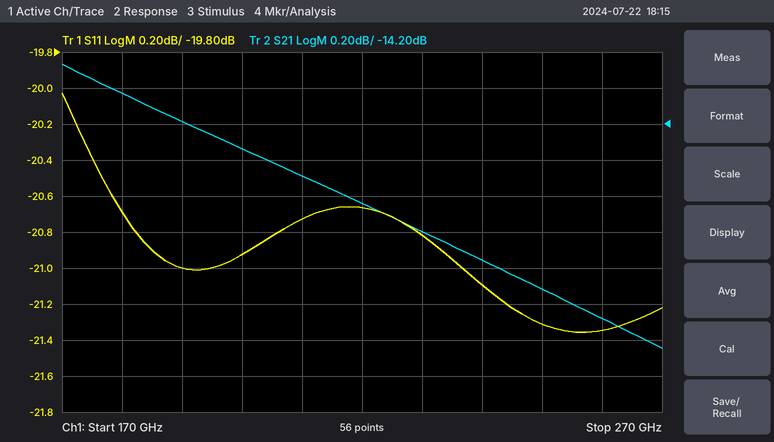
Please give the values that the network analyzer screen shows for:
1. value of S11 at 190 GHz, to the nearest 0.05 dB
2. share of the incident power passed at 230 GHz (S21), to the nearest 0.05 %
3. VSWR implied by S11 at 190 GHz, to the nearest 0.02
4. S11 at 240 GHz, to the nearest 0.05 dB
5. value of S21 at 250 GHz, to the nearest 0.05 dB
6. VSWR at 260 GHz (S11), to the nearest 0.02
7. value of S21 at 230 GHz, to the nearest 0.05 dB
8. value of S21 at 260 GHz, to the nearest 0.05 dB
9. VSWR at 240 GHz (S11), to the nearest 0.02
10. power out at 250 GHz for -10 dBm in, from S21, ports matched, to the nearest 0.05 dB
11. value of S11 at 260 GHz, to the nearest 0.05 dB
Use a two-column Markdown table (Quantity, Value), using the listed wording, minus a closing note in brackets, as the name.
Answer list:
| Quantity | Value |
|---|---|
| value of S11 at 190 GHz, to the nearest 0.05 dB | -21.00 dB |
| share of the incident power passed at 230 GHz (S21), to the nearest 0.05 % | 3.30 % |
| VSWR implied by S11 at 190 GHz, to the nearest 0.02 | 1.20 |
| S11 at 240 GHz, to the nearest 0.05 dB | -21.10 dB |
| value of S21 at 250 GHz, to the nearest 0.05 dB | -15.10 dB |
| VSWR at 260 GHz (S11), to the nearest 0.02 | 1.18 |
| value of S21 at 230 GHz, to the nearest 0.05 dB | -14.80 dB |
| value of S21 at 260 GHz, to the nearest 0.05 dB | -15.30 dB |
| VSWR at 240 GHz (S11), to the nearest 0.02 | 1.20 |
| power out at 250 GHz for -10 dBm in, from S21, ports matched, to the nearest 0.05 dB | -25.10 dBm |
| value of S11 at 260 GHz, to the nearest 0.05 dB | -21.35 dB |
